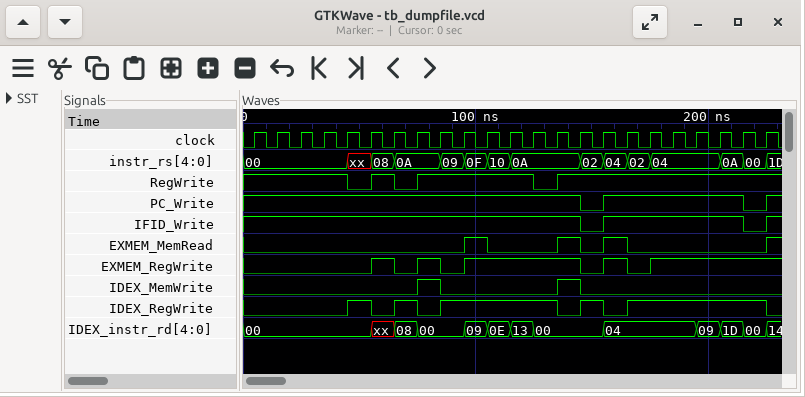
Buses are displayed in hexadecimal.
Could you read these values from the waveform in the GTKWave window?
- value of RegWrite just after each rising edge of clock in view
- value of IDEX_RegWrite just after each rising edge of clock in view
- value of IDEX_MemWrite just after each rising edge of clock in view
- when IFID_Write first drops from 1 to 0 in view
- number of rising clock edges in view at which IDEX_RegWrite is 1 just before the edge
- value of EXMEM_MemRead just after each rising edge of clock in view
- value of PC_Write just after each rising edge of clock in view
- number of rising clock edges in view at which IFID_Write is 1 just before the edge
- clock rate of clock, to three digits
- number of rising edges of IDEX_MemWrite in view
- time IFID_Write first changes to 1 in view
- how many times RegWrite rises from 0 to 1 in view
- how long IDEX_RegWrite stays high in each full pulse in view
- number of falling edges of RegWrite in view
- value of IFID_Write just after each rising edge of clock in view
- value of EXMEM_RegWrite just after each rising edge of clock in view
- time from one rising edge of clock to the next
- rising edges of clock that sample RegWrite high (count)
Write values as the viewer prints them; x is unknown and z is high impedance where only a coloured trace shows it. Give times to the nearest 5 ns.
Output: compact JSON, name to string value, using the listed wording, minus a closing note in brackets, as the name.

{"value of RegWrite just after each rising edge of clock in view": "1 1 1 1 0 1 0 1 1 1 1 1 0 1 1 1 1 1 1 1 1 1 1", "value of IDEX_RegWrite just after each rising edge of clock in view": "0 0 0 0 1 0 1 0 1 1 1 1 1 0 1 0 1 1 1 1 1 1 0", "value of IDEX_MemWrite just after each rising edge of clock in view": "0 0 0 0 0 0 0 1 0 0 0 0 0 1 0 0 0 0 0 0 0 0 0", "when IFID_Write first drops from 1 to 0 in view": "145 ns", "number of rising clock edges in view at which IDEX_RegWrite is 1 just before the edge": "14", "value of EXMEM_MemRead just after each rising edge of clock in view": "0 0 0 0 0 0 0 0 0 1 0 0 0 1 0 1 0 0 0 0 0 0 1", "value of PC_Write just after each rising edge of clock in view": "1 1 1 1 1 1 1 1 1 1 1 1 1 1 0 1 1 1 1 1 1 0 1", "number of rising clock edges in view at which IFID_Write is 1 just before the edge": "21", "clock rate of clock, to three digits": "100 MHz", "number of rising edges of IDEX_MemWrite in view": "2", "time IFID_Write first changes to 1 in view": "155 ns", "how many times RegWrite rises from 0 to 1 in view": "3", "how long IDEX_RegWrite stays high in each full pulse in view": "10 ns, 10 ns, 50 ns, 10 ns, 60 ns", "number of falling edges of RegWrite in view": "3", "value of IFID_Write just after each rising edge of clock in view": "1 1 1 1 1 1 1 1 1 1 1 1 1 1 0 1 1 1 1 1 1 0 1", "value of EXMEM_RegWrite just after each rising edge of clock in view": "0 0 0 0 0 1 0 1 0 1 1 1 1 1 0 1 0 1 1 1 1 1 1", "time from one rising edge of clock to the next": "10 ns", "rising edges of clock that sample RegWrite high": "20"}
